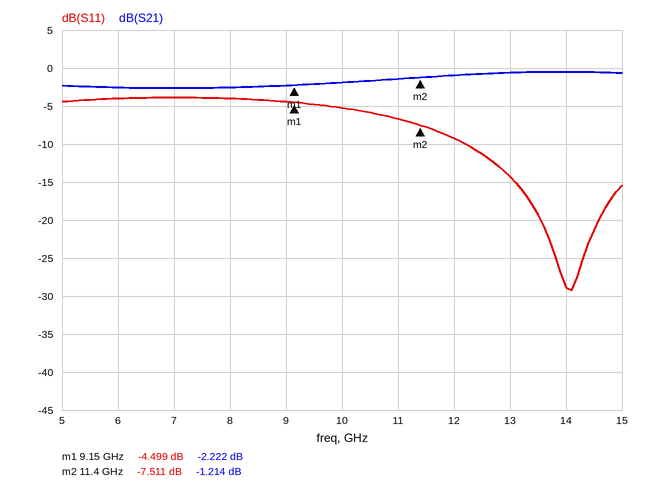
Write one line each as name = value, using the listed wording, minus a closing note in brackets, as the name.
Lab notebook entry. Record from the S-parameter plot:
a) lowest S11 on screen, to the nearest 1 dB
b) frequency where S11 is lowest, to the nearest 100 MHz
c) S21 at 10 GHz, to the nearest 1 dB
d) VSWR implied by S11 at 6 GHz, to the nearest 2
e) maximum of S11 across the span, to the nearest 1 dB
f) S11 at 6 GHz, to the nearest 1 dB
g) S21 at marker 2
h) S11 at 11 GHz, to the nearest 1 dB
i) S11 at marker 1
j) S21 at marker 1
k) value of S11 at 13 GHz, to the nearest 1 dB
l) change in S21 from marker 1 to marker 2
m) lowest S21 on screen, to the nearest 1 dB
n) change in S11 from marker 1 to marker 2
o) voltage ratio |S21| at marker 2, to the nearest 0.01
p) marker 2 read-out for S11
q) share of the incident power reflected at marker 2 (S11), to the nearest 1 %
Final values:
lowest S11 on screen, to the nearest 1 dB = -29 dB
frequency where S11 is lowest, to the nearest 100 MHz = 14.1 GHz
S21 at 10 GHz, to the nearest 1 dB = -2 dB
VSWR implied by S11 at 6 GHz, to the nearest 2 = 4
maximum of S11 across the span, to the nearest 1 dB = -4 dB
S11 at 6 GHz, to the nearest 1 dB = -4 dB
S21 at marker 2 = -1.214 dB
S11 at 11 GHz, to the nearest 1 dB = -7 dB
S11 at marker 1 = -4.499 dB
S21 at marker 1 = -2.222 dB
value of S11 at 13 GHz, to the nearest 1 dB = -14 dB
change in S21 from marker 1 to marker 2 = 1.008 dB
lowest S21 on screen, to the nearest 1 dB = -3 dB
change in S11 from marker 1 to marker 2 = -3.012 dB
voltage ratio |S21| at marker 2, to the nearest 0.01 = 0.87
marker 2 read-out for S11 = -7.511 dB
share of the incident power reflected at marker 2 (S11), to the nearest 1 % = 18 %
